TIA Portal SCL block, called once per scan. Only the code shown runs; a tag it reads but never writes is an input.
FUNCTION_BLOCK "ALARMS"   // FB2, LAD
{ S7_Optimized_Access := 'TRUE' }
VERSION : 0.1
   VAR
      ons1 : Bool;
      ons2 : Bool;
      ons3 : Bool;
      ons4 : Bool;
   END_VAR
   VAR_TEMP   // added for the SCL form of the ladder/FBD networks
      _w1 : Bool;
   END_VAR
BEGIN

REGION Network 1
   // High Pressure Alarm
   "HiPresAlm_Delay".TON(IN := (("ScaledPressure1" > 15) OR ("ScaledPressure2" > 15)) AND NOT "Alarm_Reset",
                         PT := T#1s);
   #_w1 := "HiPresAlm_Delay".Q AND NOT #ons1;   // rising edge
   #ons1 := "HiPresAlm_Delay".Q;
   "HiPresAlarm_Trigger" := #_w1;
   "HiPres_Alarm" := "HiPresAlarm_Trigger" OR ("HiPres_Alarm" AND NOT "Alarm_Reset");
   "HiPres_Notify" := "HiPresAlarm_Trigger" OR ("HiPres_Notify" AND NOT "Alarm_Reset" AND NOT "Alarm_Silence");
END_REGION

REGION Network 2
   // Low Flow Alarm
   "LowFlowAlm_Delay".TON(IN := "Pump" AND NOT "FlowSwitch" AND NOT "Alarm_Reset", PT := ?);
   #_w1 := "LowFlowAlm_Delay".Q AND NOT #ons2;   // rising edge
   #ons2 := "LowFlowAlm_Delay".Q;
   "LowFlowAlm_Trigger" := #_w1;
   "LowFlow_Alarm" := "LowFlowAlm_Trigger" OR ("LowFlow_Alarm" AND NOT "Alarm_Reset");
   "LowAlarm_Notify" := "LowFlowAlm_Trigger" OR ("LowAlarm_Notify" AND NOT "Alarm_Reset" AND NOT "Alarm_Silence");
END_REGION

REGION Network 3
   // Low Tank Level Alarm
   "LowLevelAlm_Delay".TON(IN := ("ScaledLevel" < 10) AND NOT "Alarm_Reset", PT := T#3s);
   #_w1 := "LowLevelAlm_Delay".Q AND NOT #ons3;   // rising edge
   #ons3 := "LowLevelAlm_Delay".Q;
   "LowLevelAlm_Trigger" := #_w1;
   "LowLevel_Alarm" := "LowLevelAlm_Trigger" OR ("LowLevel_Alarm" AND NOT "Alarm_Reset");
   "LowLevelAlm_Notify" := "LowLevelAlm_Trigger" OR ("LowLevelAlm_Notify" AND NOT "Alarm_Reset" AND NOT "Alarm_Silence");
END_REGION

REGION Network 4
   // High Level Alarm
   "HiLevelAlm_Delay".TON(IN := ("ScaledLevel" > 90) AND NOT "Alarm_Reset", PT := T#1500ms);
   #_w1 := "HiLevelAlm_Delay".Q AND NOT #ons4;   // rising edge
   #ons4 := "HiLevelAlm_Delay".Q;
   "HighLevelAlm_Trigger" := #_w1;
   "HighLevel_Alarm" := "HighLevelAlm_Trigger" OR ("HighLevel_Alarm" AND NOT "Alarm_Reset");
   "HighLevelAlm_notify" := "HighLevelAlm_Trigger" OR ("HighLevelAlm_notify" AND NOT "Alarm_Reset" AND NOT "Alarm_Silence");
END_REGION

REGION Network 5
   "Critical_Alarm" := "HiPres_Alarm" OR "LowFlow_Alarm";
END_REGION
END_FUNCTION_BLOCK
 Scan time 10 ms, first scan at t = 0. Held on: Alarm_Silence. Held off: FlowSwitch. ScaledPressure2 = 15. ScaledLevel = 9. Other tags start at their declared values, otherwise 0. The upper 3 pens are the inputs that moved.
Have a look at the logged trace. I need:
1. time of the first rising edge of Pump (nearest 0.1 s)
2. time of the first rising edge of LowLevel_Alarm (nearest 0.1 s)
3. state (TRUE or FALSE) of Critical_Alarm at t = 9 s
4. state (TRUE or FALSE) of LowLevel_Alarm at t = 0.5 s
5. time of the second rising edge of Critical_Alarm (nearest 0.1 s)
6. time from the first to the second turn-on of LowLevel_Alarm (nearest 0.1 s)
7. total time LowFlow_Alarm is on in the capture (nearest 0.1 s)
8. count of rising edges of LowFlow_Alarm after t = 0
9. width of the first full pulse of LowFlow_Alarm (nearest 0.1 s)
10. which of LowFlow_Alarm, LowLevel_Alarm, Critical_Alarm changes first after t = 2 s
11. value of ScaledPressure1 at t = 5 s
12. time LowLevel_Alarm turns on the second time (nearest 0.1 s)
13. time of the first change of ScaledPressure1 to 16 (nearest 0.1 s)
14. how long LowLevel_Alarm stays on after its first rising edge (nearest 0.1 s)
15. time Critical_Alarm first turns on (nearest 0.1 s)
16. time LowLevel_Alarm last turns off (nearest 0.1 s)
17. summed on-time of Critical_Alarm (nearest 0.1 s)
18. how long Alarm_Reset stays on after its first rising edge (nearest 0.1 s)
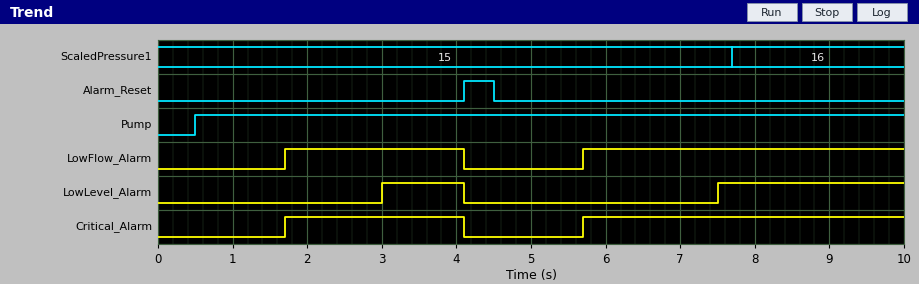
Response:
0.5 s
3.0 s
TRUE
FALSE
5.7 s
4.5 s
6.7 s
2
2.4 s
LowLevel_Alarm
15
7.5 s
7.7 s
1.1 s
1.7 s
4.1 s
6.7 s
0.4 s
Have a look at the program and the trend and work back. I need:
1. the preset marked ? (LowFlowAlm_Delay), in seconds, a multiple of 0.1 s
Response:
1.2 s
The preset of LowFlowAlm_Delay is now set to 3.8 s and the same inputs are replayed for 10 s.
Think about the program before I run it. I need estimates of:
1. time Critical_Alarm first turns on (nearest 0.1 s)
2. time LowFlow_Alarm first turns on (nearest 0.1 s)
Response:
8.3 s
8.3 s
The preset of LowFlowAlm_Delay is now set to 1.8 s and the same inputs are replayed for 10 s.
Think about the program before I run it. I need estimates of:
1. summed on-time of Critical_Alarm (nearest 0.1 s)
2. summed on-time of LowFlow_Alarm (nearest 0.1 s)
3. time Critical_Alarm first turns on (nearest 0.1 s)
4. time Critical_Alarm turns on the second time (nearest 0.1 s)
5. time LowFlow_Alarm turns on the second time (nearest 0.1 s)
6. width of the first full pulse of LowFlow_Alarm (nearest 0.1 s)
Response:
5.5 s
5.5 s
2.3 s
6.3 s
6.3 s
1.8 s
